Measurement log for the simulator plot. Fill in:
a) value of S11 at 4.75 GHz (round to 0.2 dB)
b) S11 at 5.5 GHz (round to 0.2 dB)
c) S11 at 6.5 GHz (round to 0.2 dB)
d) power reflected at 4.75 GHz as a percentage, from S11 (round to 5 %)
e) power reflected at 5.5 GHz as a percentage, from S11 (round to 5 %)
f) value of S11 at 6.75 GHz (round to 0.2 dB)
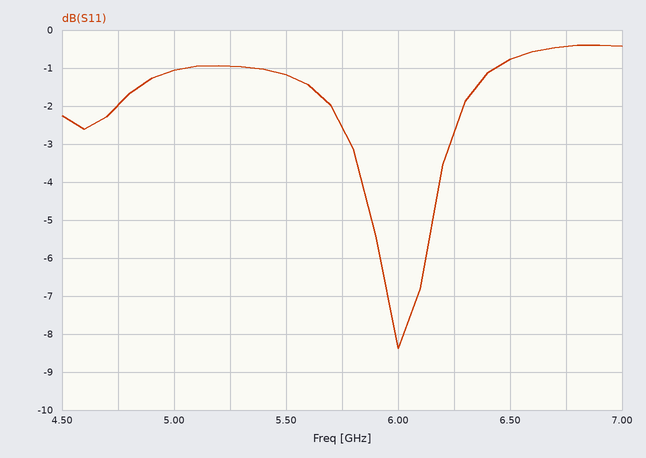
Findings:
-2.0 dB
-1.2 dB
-0.8 dB
65 %
75 %
-0.4 dB
